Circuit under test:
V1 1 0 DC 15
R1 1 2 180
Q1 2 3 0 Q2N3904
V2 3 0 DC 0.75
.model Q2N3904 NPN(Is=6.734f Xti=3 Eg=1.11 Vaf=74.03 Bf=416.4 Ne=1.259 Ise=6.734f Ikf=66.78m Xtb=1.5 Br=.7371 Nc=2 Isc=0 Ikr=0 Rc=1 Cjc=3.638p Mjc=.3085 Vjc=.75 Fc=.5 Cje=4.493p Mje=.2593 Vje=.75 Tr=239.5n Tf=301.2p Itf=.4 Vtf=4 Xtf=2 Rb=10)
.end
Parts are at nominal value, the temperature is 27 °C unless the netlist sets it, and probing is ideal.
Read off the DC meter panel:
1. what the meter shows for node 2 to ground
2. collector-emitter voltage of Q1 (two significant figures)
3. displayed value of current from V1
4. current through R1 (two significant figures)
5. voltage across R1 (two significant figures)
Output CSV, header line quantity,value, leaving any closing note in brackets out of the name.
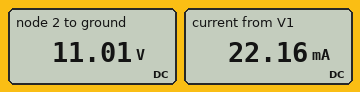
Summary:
quantity,value
what the meter shows for node 2 to ground,11.01 V
collector-emitter voltage of Q1,11 V
displayed value of current from V1,22.16 mA
current through R1,22 mA
voltage across R1,4.0 V
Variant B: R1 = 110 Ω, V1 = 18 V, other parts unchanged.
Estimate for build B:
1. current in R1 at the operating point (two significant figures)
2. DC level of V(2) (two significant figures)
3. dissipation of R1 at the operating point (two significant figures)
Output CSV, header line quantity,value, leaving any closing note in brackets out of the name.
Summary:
quantity,value
current in R1 at the operating point,23 mA
DC level of V(2),15 V
dissipation of R1 at the operating point,60 mW
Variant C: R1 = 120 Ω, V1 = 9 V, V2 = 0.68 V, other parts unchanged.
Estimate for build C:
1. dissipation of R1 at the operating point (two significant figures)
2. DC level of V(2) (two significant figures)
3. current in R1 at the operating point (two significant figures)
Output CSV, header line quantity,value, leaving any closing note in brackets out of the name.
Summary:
quantity,value
dissipation of R1 at the operating point,430 µW
DC level of V(2),8.8 V
current in R1 at the operating point,1.9 mA
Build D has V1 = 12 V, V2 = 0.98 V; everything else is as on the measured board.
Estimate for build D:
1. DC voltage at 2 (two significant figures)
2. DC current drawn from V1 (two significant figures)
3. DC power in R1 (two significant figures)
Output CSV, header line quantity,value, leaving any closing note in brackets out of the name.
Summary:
quantity,value
DC voltage at 2,140 mV
DC current drawn from V1,66 mA
DC power in R1,780 mW
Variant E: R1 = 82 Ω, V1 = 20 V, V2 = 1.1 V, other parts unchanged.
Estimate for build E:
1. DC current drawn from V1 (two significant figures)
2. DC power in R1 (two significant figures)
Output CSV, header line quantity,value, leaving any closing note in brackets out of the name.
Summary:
quantity,value
DC current drawn from V1,240 mA
DC power in R1,4.7 W
